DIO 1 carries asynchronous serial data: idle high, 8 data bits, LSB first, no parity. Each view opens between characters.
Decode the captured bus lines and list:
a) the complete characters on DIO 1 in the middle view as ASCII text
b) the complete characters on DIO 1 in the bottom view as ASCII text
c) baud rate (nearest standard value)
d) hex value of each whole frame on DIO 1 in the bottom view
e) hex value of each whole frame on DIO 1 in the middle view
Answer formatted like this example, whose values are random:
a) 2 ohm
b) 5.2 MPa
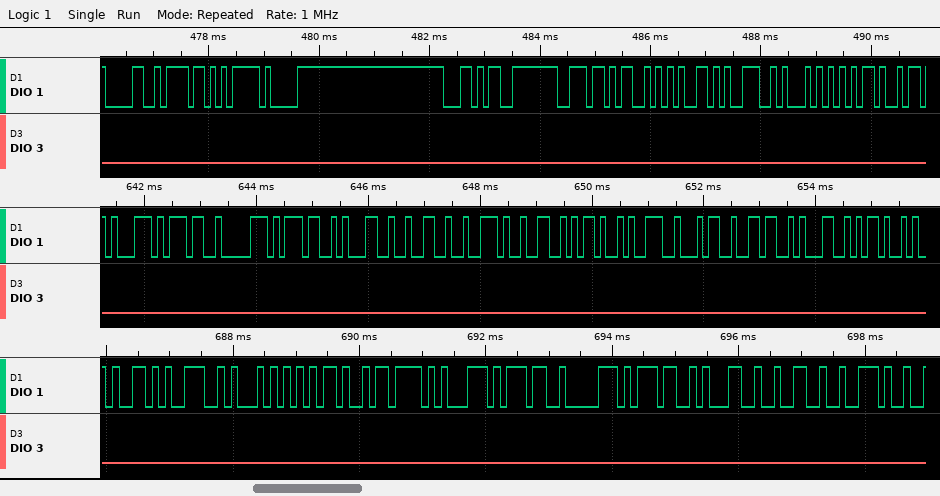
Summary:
a) "q7p712r2-9461-"
b) "YNT-{q7p712r"
c) 9600 baud
d) 59, 4E, 54, 2D, 7B, 71, 37, 70, 37, 31, 32, 72
e) 71, 37, 70, 37, 31, 32, 72, 32, 2D, 39, 34, 36, 31, 2D
